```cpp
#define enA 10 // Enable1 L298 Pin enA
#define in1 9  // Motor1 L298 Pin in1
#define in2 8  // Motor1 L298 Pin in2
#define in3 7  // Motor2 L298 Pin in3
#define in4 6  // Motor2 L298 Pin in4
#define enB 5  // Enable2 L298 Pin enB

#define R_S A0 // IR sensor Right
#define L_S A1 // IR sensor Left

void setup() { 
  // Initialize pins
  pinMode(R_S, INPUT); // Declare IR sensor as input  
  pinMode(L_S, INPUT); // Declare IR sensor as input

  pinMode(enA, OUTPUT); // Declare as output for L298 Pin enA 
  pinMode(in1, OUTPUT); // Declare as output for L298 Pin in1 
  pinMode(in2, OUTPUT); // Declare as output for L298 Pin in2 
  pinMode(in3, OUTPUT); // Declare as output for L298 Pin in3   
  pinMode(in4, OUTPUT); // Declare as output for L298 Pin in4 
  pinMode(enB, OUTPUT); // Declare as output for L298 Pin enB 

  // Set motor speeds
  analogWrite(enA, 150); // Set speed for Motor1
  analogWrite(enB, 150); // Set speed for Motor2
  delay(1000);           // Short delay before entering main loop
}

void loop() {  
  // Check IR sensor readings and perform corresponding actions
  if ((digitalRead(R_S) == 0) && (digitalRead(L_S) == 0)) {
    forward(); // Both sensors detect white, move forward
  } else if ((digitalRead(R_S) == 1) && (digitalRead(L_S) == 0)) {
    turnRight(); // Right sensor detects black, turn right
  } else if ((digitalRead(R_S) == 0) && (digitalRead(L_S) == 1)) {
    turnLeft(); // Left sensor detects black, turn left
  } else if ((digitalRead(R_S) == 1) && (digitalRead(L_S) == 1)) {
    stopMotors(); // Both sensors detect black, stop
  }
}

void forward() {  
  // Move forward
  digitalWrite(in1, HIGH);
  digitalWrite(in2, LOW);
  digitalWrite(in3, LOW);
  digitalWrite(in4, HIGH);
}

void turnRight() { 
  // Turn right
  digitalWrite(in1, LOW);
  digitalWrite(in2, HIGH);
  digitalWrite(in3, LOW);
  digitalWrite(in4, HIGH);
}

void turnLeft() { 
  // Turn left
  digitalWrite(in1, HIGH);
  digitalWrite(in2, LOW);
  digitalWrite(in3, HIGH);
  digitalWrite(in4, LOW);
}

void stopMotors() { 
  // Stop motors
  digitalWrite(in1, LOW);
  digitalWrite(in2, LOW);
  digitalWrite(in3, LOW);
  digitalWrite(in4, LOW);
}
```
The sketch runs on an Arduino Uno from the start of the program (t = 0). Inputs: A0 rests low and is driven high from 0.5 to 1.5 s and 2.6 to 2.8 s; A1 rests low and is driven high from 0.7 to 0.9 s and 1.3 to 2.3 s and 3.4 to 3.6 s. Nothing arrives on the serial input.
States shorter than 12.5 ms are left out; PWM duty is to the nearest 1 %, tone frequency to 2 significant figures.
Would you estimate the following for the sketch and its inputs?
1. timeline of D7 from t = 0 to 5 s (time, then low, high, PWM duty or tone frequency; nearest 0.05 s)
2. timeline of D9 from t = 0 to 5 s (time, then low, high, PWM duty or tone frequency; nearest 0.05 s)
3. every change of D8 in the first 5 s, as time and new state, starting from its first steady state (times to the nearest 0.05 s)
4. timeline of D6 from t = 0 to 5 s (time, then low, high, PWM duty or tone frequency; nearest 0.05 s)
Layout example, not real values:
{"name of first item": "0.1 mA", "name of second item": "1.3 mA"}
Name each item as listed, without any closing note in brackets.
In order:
{"timeline of D7 from t = 0 to 5 s": "0 s low; 1.5 s high; 2.3 s low; 3.4 s high; 3.6 s low", "timeline of D9 from t = 0 to 5 s": "0 s low; 1.5 s high; 2.6 s low; 2.8 s high", "every change of D8 in the first 5 s, as time and new state, starting from its first steady state": "0 s low; 1 s high; 1.3 s low; 2.6 s high; 2.8 s low", "timeline of D6 from t = 0 to 5 s": "0 s low; 1 s high; 1.3 s low; 2.3 s high; 3.4 s low; 3.6 s high"}
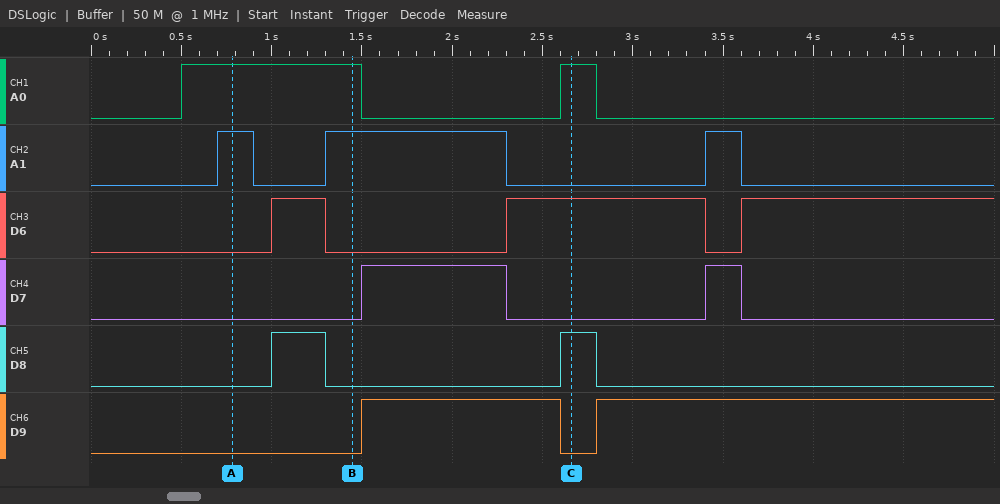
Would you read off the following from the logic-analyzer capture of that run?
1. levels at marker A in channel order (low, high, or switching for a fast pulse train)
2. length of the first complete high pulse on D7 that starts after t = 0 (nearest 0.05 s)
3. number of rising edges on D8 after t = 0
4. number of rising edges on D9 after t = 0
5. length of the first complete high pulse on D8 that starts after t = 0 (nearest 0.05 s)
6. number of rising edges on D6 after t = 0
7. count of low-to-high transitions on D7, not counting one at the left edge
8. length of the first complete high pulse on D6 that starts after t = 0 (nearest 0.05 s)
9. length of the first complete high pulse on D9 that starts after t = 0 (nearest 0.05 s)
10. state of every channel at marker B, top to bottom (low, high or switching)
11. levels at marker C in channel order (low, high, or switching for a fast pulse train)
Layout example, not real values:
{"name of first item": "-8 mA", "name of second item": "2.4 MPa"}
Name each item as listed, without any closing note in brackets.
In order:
{"levels at marker A in channel order": "A0 high, A1 high, D6 low, D7 low, D8 low, D9 low", "length of the first complete high pulse on D7 that starts after t = 0": "0.80 s", "number of rising edges on D8 after t = 0": "2", "number of rising edges on D9 after t = 0": "2", "length of the first complete high pulse on D8 that starts after t = 0": "0.30 s", "number of rising edges on D6 after t = 0": "3", "count of low-to-high transitions on D7, not counting one at the left edge": "2", "length of the first complete high pulse on D6 that starts after t = 0": "0.30 s", "length of the first complete high pulse on D9 that starts after t = 0": "1.10 s", "state of every channel at marker B, top to bottom": "A0 high, A1 high, D6 low, D7 low, D8 low, D9 low", "levels at marker C in channel order": "A0 high, A1 low, D6 high, D7 low, D8 high, D9 low"}
